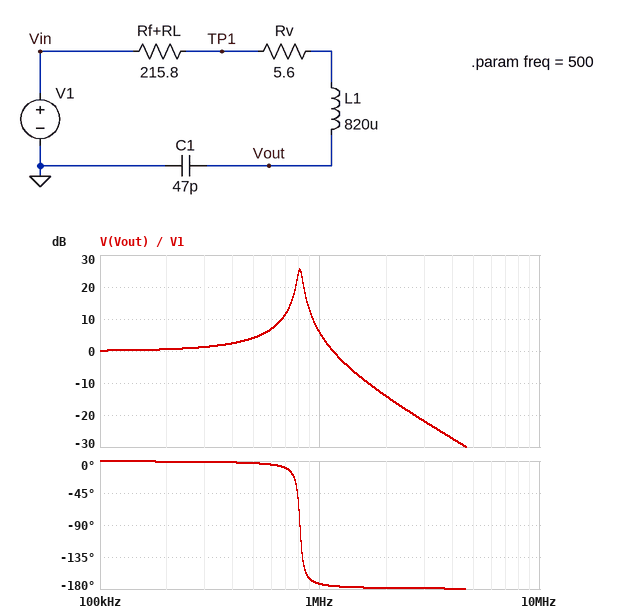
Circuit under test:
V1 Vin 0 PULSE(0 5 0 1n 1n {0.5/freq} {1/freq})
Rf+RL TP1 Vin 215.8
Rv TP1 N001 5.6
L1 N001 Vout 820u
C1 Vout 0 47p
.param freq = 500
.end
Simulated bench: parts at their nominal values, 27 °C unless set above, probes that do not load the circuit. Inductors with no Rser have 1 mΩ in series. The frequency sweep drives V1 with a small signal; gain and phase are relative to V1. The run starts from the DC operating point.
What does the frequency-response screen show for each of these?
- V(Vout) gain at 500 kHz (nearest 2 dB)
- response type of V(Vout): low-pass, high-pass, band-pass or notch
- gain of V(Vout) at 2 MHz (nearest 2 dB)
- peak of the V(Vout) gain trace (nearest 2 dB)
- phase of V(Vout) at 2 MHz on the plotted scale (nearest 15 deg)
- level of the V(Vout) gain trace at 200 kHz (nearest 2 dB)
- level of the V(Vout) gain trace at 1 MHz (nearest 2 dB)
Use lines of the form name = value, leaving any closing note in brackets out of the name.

V(Vout) gain at 500 kHz = 4 dB
response type of V(Vout): low-pass, high-pass, band-pass or notch = low-pass
gain of V(Vout) at 2 MHz = -14 dB
peak of the V(Vout) gain trace = 26 dB
phase of V(Vout) at 2 MHz on the plotted scale = -180 deg
level of the V(Vout) gain trace at 200 kHz = 0 dB
level of the V(Vout) gain trace at 1 MHz = 6 dB
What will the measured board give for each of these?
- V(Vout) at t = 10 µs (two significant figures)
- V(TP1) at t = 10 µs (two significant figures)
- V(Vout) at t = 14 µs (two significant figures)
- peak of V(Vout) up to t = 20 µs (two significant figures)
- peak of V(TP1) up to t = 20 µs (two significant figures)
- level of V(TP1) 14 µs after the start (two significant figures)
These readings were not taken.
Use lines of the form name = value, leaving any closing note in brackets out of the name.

V(Vout) at t = 10 µs = 3.9 V
V(TP1) at t = 10 µs = 5.0 V
V(Vout) at t = 14 µs = 5.4 V
peak of V(Vout) up to t = 20 µs = 9.6 V
peak of V(TP1) up to t = 20 µs = 5.2 V
level of V(TP1) 14 µs after the start = 5.0 V
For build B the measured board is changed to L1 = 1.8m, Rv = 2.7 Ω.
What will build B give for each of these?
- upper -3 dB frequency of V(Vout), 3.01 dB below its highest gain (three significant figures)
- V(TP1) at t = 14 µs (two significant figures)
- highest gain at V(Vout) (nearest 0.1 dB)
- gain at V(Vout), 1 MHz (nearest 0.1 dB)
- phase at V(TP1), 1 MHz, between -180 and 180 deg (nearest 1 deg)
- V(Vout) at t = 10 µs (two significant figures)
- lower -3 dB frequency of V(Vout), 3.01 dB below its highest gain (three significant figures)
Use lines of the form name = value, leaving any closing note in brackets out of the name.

upper -3 dB frequency of V(Vout), 3.01 dB below its highest gain = 557 kHz
V(TP1) at t = 14 µs = 5.1 V
highest gain at V(Vout) = 29.0 dB
gain at V(Vout), 1 MHz = -7.4 dB
phase at V(TP1), 1 MHz, between -180 and 180 deg = 2 deg
V(Vout) at t = 10 µs = 7.7 V
lower -3 dB frequency of V(Vout), 3.01 dB below its highest gain = 537 kHz
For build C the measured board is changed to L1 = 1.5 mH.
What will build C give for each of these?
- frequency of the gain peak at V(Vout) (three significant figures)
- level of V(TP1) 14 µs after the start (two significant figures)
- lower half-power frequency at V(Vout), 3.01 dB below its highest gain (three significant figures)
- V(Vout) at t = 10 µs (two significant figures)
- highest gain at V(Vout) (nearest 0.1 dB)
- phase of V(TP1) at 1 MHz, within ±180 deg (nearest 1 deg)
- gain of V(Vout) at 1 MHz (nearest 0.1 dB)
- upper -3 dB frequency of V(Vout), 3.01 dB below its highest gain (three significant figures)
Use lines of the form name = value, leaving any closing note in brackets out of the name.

frequency of the gain peak at V(Vout) = 599 kHz
level of V(TP1) 14 µs after the start = 5.0 V
lower half-power frequency at V(Vout), 3.01 dB below its highest gain = 587 kHz
V(Vout) at t = 10 µs = 2.6 V
highest gain at V(Vout) = 28.1 dB
phase of V(TP1) at 1 MHz, within ±180 deg = 2 deg
gain of V(Vout) at 1 MHz = -5.0 dB
upper -3 dB frequency of V(Vout), 3.01 dB below its highest gain = 611 kHz
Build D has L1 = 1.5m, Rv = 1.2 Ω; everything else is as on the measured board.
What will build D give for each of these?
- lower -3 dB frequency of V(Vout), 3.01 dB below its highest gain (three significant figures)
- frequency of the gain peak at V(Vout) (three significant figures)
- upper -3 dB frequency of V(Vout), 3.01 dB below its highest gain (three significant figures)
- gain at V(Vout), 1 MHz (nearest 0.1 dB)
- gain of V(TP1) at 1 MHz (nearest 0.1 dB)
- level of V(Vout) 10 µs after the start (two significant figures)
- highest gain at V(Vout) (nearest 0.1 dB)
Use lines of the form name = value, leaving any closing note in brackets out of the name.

lower -3 dB frequency of V(Vout), 3.01 dB below its highest gain = 588 kHz
frequency of the gain peak at V(Vout) = 599 kHz
upper -3 dB frequency of V(Vout), 3.01 dB below its highest gain = 611 kHz
gain at V(Vout), 1 MHz = -5.0 dB
gain of V(TP1) at 1 MHz = 0 dB
level of V(Vout) 10 µs after the start = 2.6 V
highest gain at V(Vout) = 28.3 dB
